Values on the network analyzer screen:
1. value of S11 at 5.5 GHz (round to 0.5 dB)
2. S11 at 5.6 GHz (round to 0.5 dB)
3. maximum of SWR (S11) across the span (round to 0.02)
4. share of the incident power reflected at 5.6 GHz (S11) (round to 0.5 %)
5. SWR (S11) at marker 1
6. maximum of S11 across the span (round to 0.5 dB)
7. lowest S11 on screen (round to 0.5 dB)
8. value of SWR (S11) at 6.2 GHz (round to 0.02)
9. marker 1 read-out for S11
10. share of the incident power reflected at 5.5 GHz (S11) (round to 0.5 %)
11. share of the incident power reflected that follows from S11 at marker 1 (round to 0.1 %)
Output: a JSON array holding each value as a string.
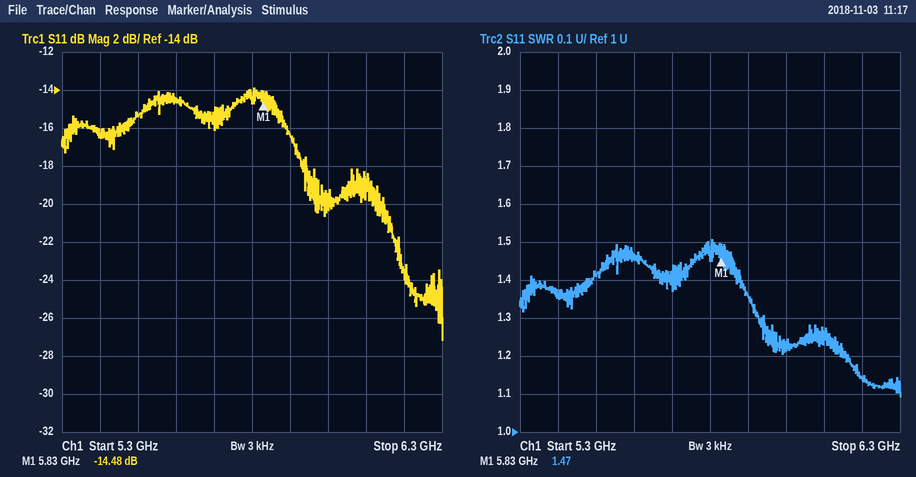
["-15.5 dB", "-14.5 dB", "1.50", "3.5 %", "1.47", "-14.0 dB", "-27.0 dB", "1.14", "-14.48 dB", "3.0 %", "3.6 %"]
